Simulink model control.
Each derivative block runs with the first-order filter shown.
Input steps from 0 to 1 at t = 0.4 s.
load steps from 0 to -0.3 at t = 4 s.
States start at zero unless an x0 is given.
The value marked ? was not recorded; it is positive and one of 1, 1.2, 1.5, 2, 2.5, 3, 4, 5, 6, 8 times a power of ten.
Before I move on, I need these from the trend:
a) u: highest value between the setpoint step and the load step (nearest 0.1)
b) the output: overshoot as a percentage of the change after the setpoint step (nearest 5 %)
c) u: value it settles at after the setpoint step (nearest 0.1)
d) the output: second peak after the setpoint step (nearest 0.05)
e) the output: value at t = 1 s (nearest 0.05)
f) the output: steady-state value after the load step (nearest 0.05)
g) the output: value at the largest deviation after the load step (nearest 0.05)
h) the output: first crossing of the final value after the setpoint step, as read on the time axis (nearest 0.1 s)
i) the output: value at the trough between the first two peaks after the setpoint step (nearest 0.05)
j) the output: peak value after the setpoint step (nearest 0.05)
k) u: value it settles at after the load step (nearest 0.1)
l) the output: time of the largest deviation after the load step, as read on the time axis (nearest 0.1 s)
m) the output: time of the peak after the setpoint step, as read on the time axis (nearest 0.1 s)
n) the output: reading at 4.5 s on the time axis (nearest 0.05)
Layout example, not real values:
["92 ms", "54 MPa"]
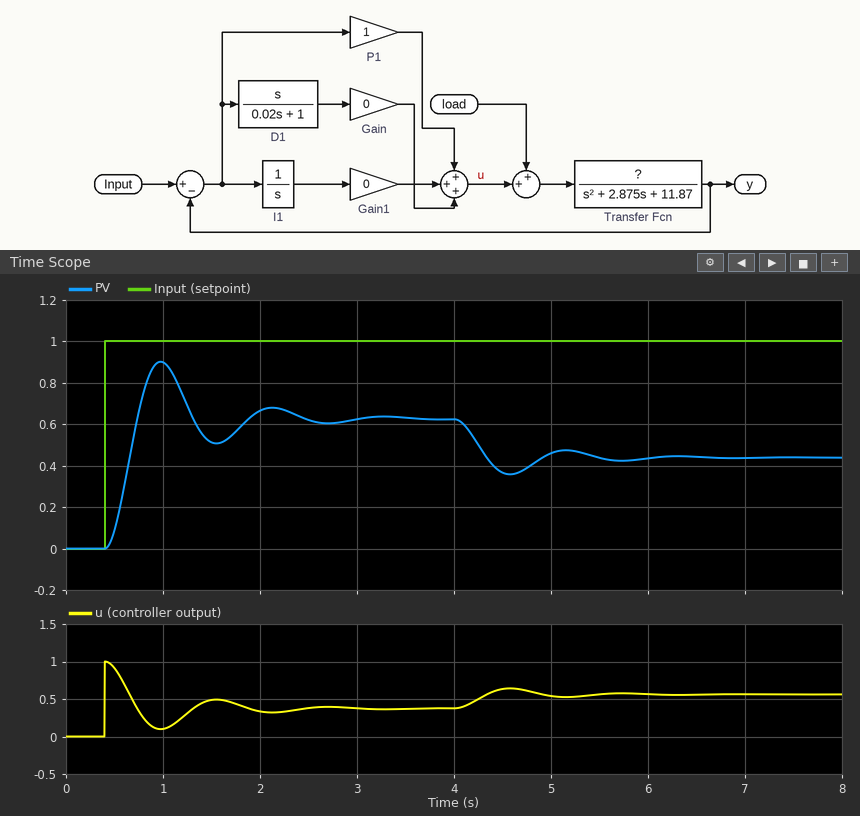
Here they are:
["1.0", "45 %", "0.4", "0.70", "0.90", "0.45", "0.35", "0.7 s", "0.50", "0.90", "0.6", "4.6 s", "1.0 s", "0.35"]
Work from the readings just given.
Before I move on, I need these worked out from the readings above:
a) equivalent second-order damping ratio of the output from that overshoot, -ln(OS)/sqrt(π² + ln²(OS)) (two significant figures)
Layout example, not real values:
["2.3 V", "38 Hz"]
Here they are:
["0.25"]
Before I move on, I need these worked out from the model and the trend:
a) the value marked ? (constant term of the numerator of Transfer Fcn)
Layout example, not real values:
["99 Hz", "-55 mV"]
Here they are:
["20"]
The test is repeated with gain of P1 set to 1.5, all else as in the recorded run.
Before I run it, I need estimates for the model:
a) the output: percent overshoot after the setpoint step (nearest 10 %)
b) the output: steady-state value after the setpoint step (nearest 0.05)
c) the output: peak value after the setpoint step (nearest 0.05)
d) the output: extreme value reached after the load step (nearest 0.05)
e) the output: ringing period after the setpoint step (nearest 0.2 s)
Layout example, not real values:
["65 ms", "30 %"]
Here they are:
["50 %", "0.70", "1.05", "0.50", "1.0 s"]
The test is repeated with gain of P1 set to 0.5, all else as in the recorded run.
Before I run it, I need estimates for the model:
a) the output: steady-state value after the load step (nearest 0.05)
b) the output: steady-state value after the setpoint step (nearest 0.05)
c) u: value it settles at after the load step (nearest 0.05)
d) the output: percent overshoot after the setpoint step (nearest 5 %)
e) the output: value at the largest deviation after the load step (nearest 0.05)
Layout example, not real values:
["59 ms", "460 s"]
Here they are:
["0.20", "0.45", "0.40", "35 %", "0.10"]
